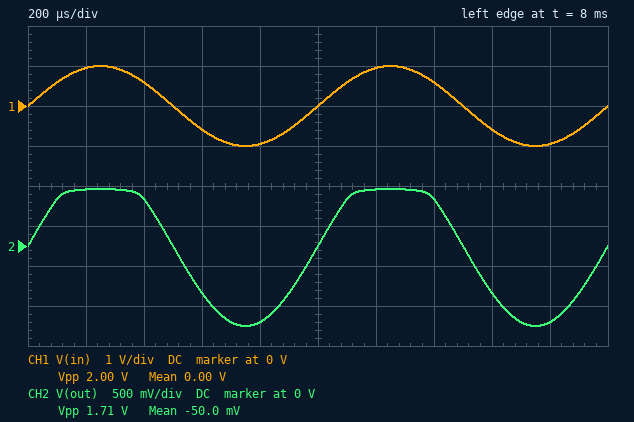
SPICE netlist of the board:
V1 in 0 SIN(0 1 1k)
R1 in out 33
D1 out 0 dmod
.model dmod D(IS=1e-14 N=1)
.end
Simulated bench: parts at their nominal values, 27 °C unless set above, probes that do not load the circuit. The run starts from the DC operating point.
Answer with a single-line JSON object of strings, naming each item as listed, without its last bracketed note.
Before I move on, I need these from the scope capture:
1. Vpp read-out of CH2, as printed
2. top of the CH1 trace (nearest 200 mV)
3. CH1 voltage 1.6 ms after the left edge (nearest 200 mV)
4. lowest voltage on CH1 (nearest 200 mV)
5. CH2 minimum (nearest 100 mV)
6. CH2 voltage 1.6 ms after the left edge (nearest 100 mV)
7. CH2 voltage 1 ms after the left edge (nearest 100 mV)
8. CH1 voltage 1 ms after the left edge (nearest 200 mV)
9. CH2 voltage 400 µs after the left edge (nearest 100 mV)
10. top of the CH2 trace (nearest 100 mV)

{"Vpp read-out of CH2, as printed": "1.71 V", "top of the CH1 trace": "1.0 V", "CH1 voltage 1.6 ms after the left edge": "-600 mV", "lowest voltage on CH1": "-1.0 V", "CH2 minimum": "-1.0 V", "CH2 voltage 1.6 ms after the left edge": "-600 mV", "CH2 voltage 1 ms after the left edge": "0 V", "CH1 voltage 1 ms after the left edge": "0 V", "CH2 voltage 400 µs after the left edge": "600 mV", "top of the CH2 trace": "700 mV"}
